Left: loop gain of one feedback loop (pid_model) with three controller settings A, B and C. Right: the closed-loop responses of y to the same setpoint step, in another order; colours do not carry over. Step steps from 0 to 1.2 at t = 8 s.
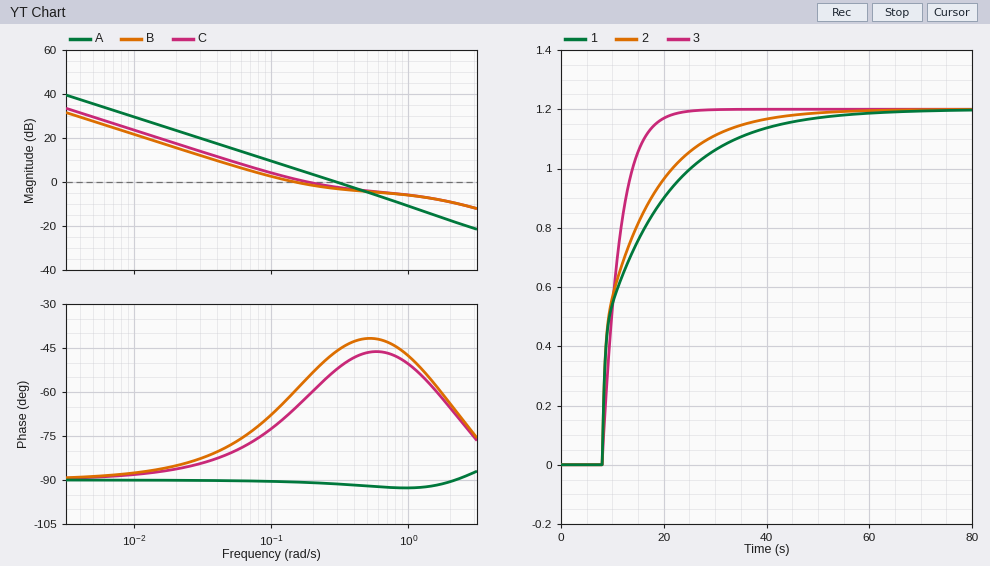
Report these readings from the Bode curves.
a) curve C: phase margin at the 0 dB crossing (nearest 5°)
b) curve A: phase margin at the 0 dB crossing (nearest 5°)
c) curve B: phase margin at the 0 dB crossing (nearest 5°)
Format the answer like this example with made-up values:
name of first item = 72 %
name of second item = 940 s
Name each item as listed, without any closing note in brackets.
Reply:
curve C: phase margin at the 0 dB crossing = 120°
curve A: phase margin at the 0 dB crossing = 90°
curve B: phase margin at the 0 dB crossing = 120°
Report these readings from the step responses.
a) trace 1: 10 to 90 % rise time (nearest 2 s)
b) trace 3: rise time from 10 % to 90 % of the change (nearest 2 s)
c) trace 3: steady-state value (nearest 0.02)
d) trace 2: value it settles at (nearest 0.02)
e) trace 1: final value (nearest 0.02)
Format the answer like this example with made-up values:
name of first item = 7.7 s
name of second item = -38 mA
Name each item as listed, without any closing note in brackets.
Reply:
trace 1: 10 to 90 % rise time = 24 s
trace 3: rise time from 10 % to 90 % of the change = 8 s
trace 3: steady-state value = 1.20
trace 2: value it settles at = 1.20
trace 1: final value = 1.20
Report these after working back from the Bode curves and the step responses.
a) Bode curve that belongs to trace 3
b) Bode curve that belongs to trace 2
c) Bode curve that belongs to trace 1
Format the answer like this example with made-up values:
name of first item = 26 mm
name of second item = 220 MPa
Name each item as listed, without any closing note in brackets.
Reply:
Bode curve that belongs to trace 3 = A
Bode curve that belongs to trace 2 = C
Bode curve that belongs to trace 1 = B
